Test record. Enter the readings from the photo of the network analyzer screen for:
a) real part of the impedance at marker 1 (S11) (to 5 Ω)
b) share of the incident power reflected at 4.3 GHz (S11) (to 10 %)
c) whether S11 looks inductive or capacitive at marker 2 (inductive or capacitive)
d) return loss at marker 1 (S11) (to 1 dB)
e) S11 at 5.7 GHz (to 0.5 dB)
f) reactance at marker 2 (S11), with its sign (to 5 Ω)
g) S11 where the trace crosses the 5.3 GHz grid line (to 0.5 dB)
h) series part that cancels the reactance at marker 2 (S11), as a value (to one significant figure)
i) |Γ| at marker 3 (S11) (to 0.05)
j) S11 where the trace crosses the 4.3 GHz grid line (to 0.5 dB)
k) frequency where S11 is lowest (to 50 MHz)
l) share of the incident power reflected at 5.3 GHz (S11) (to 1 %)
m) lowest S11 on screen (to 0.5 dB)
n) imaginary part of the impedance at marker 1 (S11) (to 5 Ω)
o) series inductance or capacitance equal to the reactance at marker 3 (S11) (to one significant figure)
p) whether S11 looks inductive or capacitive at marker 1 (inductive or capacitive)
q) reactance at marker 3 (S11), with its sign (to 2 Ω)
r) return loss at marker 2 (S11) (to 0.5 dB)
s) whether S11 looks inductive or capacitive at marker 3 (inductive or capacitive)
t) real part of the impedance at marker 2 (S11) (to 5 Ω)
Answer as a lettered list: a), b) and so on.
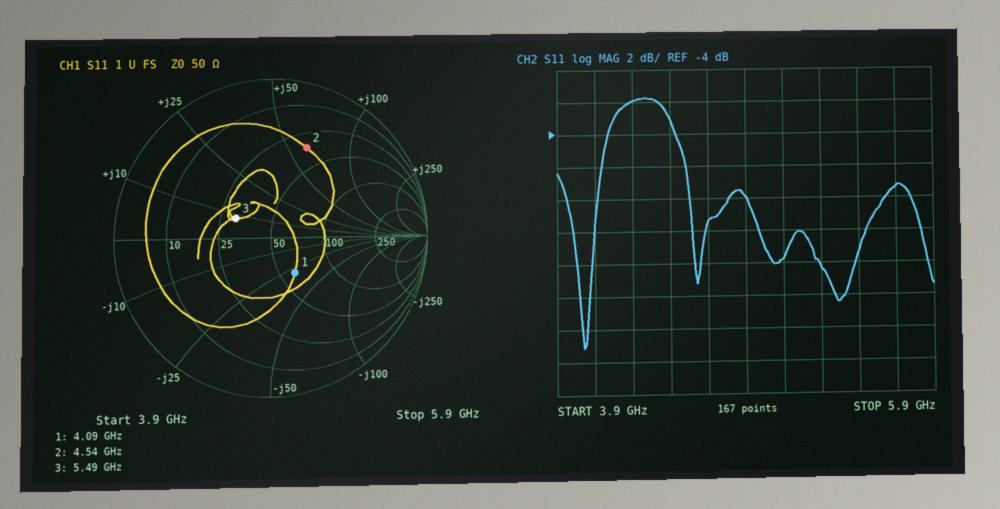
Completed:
a) 60 Ω
b) 60 %
c) inductive
d) 11 dB
e) -7.5 dB
f) +60 Ω
g) -12.5 dB
h) 600 fF
i) 0.25
j) -2.0 dB
k) 4.05 GHz
l) 6 %
m) -17.0 dB
n) -30 Ω
o) 200 pH
p) capacitive
q) +8 Ω
r) 4.5 dB
s) inductive
t) 35 Ω
